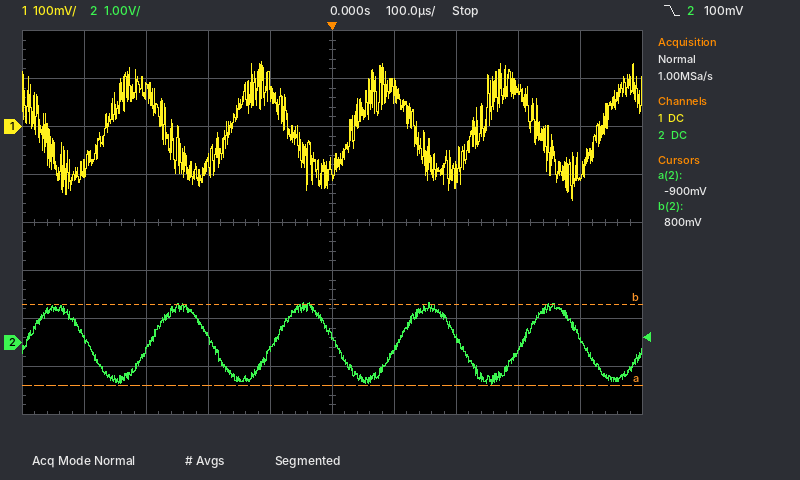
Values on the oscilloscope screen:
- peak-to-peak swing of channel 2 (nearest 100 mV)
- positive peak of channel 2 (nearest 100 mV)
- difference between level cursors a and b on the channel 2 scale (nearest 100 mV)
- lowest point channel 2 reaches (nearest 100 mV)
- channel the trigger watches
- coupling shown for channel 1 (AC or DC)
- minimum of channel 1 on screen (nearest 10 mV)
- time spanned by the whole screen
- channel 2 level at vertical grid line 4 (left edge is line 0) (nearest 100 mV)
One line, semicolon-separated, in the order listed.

1.7 V; 800 mV; 1.7 V; -900 mV; channel 2; DC; -150 mV; 1 ms; -100 mV
